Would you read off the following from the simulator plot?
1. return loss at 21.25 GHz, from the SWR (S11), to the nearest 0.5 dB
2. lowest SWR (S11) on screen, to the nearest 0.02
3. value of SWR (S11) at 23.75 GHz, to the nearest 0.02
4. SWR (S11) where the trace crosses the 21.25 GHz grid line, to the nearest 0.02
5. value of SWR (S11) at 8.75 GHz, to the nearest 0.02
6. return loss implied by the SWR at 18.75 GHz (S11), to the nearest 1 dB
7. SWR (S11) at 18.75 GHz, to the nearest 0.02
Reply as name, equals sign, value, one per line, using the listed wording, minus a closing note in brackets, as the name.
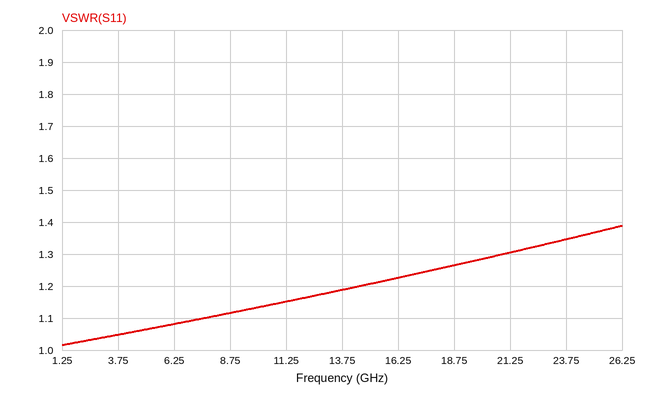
return loss at 21.25 GHz, from the SWR (S11), to the nearest 0.5 dB = 17.5 dB
lowest SWR (S11) on screen, to the nearest 0.02 = 1.02
value of SWR (S11) at 23.75 GHz, to the nearest 0.02 = 1.34
SWR (S11) where the trace crosses the 21.25 GHz grid line, to the nearest 0.02 = 1.30
value of SWR (S11) at 8.75 GHz, to the nearest 0.02 = 1.12
return loss implied by the SWR at 18.75 GHz (S11), to the nearest 1 dB = 19 dB
SWR (S11) at 18.75 GHz, to the nearest 0.02 = 1.26
